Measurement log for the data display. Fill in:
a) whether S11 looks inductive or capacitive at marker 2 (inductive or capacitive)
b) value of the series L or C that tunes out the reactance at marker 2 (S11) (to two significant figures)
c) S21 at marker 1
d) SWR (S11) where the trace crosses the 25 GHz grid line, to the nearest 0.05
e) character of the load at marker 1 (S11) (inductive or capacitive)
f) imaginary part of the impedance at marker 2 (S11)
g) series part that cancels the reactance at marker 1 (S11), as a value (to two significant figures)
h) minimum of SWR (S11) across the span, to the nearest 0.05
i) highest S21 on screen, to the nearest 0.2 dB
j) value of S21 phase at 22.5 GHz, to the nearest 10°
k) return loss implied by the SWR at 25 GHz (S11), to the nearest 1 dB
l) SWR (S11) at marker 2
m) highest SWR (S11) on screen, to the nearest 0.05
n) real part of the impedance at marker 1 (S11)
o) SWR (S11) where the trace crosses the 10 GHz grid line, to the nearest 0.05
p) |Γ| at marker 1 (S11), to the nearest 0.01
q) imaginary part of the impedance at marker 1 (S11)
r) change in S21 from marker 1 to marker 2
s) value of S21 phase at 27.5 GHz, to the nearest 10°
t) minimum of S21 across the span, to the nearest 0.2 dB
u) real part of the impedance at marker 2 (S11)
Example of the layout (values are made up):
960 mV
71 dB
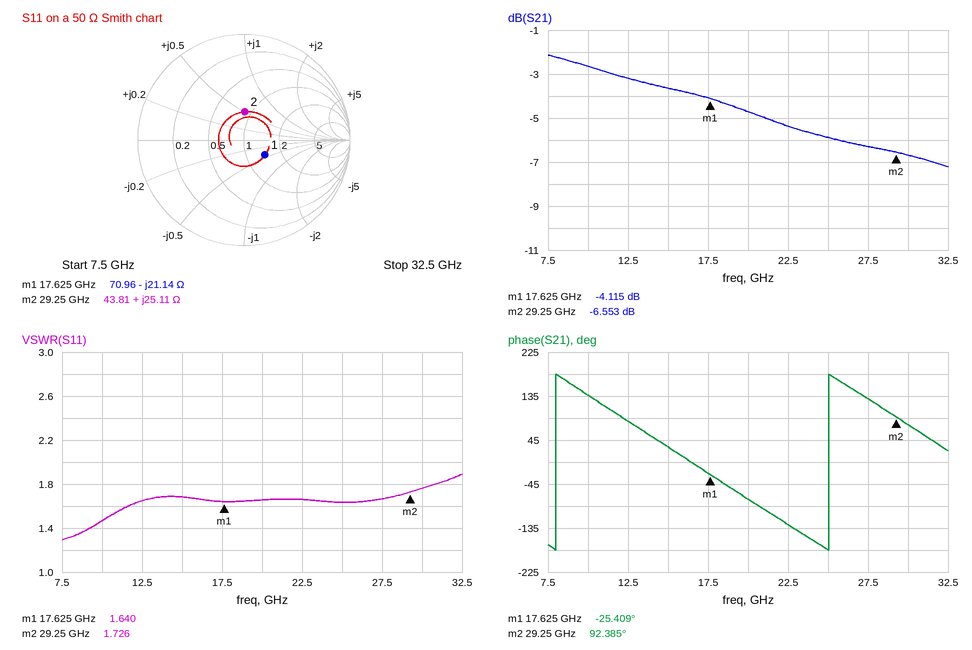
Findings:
inductive
220 fF
-4.115 dB
1.65
capacitive
+25.11 Ω
190 pH
1.30
-2.2 dB
-130°
12 dB
1.726
1.90
70.96 Ω
1.45
0.24
-21.14 Ω
-2.438 dB
130°
-7.2 dB
43.81 Ω
